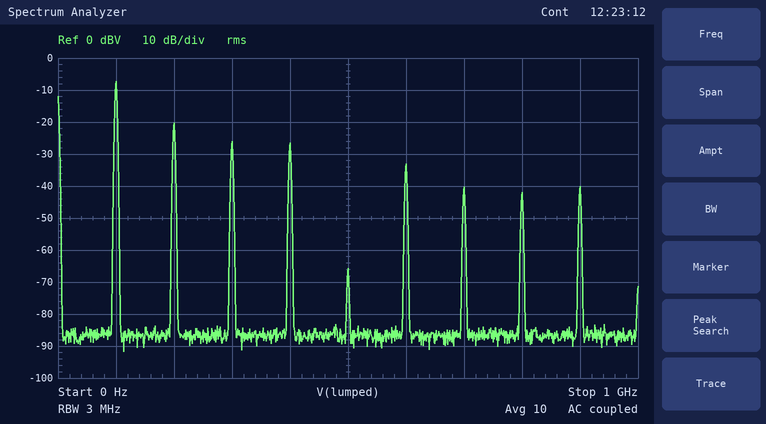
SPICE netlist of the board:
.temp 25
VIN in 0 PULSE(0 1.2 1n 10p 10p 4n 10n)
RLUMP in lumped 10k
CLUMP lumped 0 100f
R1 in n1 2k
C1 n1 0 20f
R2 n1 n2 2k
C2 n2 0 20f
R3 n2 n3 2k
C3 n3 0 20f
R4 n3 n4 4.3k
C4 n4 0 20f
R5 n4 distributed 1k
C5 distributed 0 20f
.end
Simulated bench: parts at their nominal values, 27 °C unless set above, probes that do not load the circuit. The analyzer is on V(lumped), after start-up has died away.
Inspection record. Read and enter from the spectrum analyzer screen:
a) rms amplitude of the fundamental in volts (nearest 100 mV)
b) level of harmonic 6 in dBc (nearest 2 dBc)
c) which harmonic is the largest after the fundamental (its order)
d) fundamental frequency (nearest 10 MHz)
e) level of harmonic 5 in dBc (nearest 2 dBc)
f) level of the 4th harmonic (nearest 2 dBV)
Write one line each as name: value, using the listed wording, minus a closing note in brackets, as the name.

rms amplitude of the fundamental in volts: 400 mV
level of harmonic 6 in dBc: -26 dBc
which harmonic is the largest after the fundamental: 2
fundamental frequency: 100 MHz
level of harmonic 5 in dBc: -58 dBc
level of the 4th harmonic: -26 dBV
